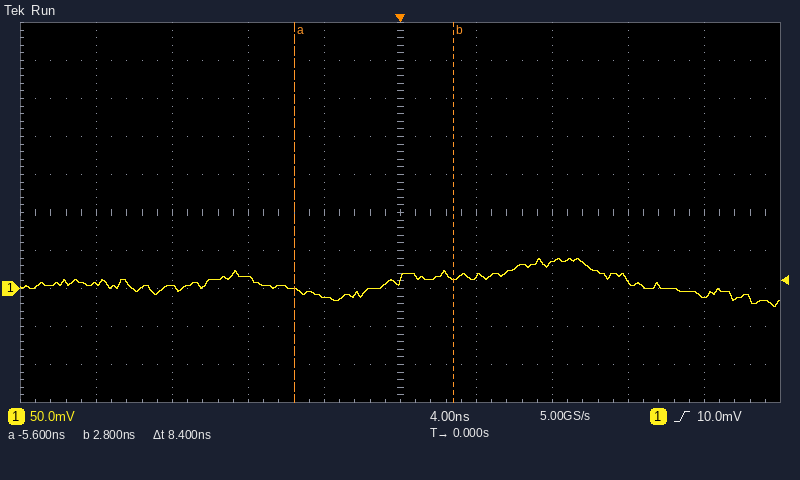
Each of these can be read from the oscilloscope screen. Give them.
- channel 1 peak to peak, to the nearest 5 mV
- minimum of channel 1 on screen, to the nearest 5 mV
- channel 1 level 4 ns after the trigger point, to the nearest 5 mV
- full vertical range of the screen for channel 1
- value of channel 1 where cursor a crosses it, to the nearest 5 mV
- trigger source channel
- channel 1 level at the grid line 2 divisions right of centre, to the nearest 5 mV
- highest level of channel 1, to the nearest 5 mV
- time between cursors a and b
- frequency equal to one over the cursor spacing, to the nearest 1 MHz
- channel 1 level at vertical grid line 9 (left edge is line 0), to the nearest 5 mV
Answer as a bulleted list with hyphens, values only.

- 65 mV
- -25 mV
- 15 mV
- 500 mV
- 0 mV
- channel 1
- 35 mV
- 40 mV
- 8.4 ns
- 119 MHz
- -10 mV
